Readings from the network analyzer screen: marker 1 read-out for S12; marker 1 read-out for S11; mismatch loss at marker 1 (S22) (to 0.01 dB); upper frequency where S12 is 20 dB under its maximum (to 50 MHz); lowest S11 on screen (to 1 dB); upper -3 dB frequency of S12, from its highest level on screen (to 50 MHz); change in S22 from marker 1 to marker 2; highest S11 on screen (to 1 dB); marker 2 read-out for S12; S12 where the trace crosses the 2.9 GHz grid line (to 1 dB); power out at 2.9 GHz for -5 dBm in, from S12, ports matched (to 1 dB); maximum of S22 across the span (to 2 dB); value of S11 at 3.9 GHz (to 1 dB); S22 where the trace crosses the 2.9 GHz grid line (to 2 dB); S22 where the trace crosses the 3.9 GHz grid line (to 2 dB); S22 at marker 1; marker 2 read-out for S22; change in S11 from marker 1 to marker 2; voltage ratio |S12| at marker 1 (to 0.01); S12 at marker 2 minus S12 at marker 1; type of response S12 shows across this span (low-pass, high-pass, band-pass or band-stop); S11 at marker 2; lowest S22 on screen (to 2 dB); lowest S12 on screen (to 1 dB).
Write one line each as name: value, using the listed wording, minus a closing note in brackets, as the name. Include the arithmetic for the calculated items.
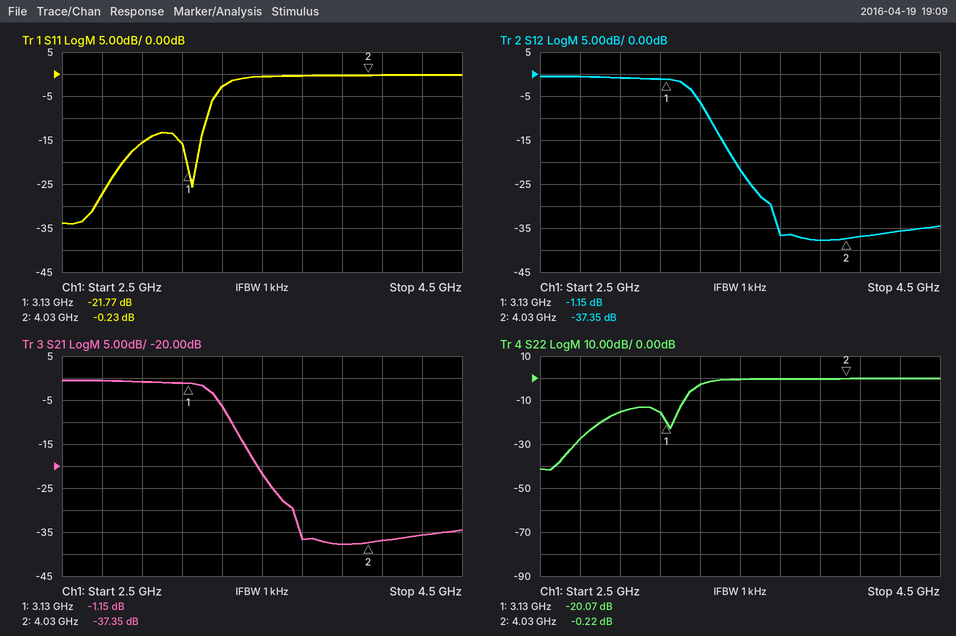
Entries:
marker 1 read-out for S12: -1.15 dB
marker 1 read-out for S11: -21.77 dB
mismatch loss at marker 1 (S22): −10 log10(1 − 10^(-20.07/10)) ≈ 0.04 dB
upper frequency where S12 is 20 dB under its maximum: 3.50 GHz
lowest S11 on screen: -34 dB
upper -3 dB frequency of S12, from its highest level on screen: 3.25 GHz
change in S22 from marker 1 to marker 2: -0.22 − (-20.07) = 19.85 dB
highest S11 on screen: 0 dB
marker 2 read-out for S12: -37.35 dB
S12 where the trace crosses the 2.9 GHz grid line: -1 dB
power out at 2.9 GHz for -5 dBm in, from S12, ports matched: -5 dBm + (-1 dB) = -6 dBm
maximum of S22 across the span: 0 dB
value of S11 at 3.9 GHz: 0 dB
S22 where the trace crosses the 2.9 GHz grid line: -16 dB
S22 where the trace crosses the 3.9 GHz grid line: 0 dB
S22 at marker 1: -20.07 dB
marker 2 read-out for S22: -0.22 dB
change in S11 from marker 1 to marker 2: -0.23 − (-21.77) = 21.54 dB
voltage ratio |S12| at marker 1: 10^(-1.15/20) ≈ 0.88
S12 at marker 2 minus S12 at marker 1: -37.35 − (-1.15) = -36.20 dB
type of response S12 shows across this span: low-pass
S11 at marker 2: -0.23 dB
lowest S22 on screen: -42 dB
lowest S12 on screen: -38 dB
